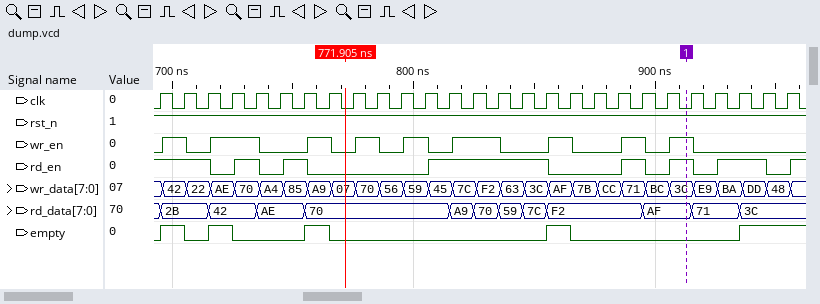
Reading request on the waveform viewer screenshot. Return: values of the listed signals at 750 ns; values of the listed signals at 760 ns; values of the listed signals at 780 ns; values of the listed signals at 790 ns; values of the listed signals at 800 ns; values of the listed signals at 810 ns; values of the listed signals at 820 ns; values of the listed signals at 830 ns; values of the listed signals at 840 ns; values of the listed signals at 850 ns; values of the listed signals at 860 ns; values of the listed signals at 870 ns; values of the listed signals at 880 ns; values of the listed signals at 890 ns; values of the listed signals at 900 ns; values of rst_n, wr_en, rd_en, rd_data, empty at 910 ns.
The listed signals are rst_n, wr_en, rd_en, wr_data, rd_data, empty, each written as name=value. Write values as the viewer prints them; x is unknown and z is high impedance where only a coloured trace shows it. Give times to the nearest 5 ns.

rst_n=1, wr_en=0, rd_en=1, wr_data=85, rd_data=AE, empty=0
rst_n=1, wr_en=1, rd_en=0, wr_data=A9, rd_data=70, empty=1
rst_n=1, wr_en=1, rd_en=0, wr_data=70, rd_data=70, empty=0
rst_n=1, wr_en=0, rd_en=0, wr_data=56, rd_data=70, empty=0
rst_n=1, wr_en=1, rd_en=0, wr_data=59, rd_data=70, empty=0
rst_n=1, wr_en=0, rd_en=1, wr_data=45, rd_data=70, empty=0
rst_n=1, wr_en=1, rd_en=1, wr_data=7C, rd_data=A9, empty=0
rst_n=1, wr_en=1, rd_en=1, wr_data=F2, rd_data=70, empty=0
rst_n=1, wr_en=0, rd_en=1, wr_data=63, rd_data=59, empty=0
rst_n=1, wr_en=0, rd_en=1, wr_data=3C, rd_data=7C, empty=0
rst_n=1, wr_en=1, rd_en=0, wr_data=AF, rd_data=F2, empty=1
rst_n=1, wr_en=0, rd_en=0, wr_data=7B, rd_data=F2, empty=0
rst_n=1, wr_en=0, rd_en=0, wr_data=CC, rd_data=F2, empty=0
rst_n=1, wr_en=1, rd_en=1, wr_data=71, rd_data=F2, empty=0
rst_n=1, wr_en=0, rd_en=0, wr_data=BC, rd_data=AF, empty=0
rst_n=1, wr_en=1, rd_en=1, rd_data=AF, empty=0
